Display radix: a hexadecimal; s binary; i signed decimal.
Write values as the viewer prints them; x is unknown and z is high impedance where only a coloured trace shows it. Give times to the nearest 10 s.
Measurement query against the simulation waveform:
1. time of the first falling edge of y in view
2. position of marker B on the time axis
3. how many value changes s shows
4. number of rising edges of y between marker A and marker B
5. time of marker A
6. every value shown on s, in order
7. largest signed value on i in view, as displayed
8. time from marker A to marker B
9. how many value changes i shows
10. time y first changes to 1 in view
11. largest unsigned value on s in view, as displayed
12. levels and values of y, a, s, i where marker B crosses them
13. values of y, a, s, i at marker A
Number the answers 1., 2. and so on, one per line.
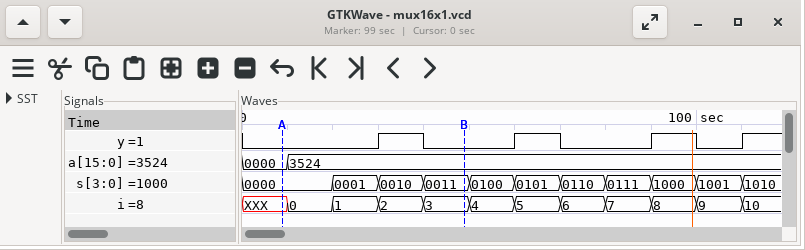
1. 40 s
2. 50 s
3. 10
4. 1
5. 10 s
6. 0000, 0001, 0010, 0011, 0100, 0101, 0110, 0111, 1000, 1001, 1010
7. 10
8. 40 s
9. 11
10. 30 s
11. 1010
12. y=0, a=3524, s=0011, i=3
13. y=0, a=0000, s=0000, i=XXX
